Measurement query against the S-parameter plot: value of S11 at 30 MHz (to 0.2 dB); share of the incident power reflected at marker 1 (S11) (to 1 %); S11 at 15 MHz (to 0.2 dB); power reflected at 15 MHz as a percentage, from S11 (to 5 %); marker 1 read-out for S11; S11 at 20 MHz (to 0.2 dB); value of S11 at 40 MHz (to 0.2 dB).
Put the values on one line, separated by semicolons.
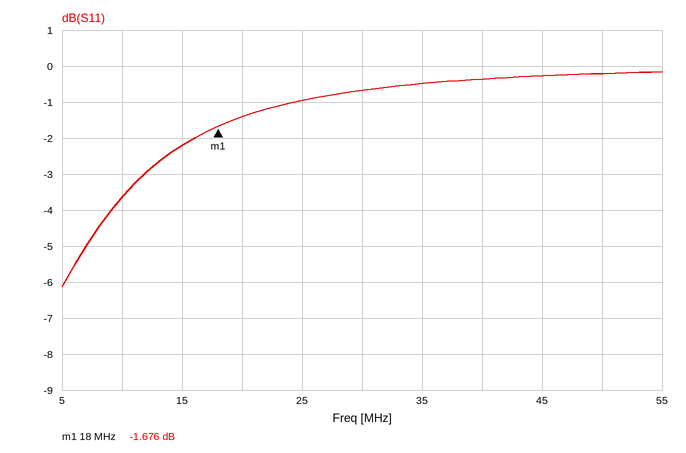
-0.6 dB; 68 %; -2.2 dB; 60 %; -1.676 dB; -1.4 dB; -0.4 dB
